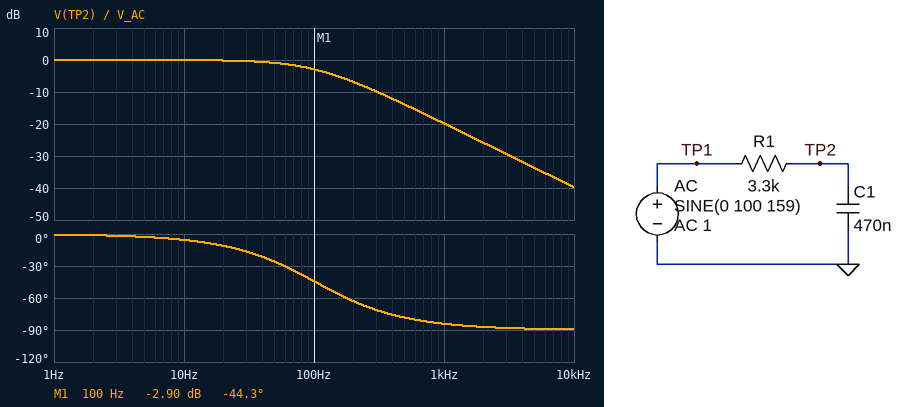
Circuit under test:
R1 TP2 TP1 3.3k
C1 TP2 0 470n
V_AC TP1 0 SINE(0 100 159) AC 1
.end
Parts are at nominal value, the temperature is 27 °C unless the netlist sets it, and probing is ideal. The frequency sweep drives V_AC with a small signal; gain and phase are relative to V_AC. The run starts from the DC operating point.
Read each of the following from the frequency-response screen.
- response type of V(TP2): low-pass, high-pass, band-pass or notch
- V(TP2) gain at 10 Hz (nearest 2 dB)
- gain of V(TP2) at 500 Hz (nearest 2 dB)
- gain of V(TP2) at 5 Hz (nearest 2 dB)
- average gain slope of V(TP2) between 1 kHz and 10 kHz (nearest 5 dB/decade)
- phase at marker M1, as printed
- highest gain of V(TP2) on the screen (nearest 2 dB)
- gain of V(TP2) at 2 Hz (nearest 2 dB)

low-pass
0 dB
-14 dB
0 dB
-20 dB/decade
-44.3 deg
0 dB
0 dB
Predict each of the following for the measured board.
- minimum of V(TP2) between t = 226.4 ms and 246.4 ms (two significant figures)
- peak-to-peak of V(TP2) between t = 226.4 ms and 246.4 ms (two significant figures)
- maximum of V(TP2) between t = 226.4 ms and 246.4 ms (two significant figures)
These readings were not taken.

-54 V
110 V
54 V
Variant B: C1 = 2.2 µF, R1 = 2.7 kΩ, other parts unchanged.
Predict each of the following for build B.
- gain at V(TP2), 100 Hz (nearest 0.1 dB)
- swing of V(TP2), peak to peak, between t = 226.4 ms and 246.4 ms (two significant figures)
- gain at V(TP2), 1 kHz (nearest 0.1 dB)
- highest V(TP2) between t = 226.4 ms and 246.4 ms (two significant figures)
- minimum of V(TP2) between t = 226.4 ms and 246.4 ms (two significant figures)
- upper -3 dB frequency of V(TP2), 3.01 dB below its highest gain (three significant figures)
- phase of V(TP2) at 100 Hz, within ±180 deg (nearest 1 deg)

-11.7 dB
33 V
-31.4 dB
17 V
-17 V
26.8 Hz
-75 deg
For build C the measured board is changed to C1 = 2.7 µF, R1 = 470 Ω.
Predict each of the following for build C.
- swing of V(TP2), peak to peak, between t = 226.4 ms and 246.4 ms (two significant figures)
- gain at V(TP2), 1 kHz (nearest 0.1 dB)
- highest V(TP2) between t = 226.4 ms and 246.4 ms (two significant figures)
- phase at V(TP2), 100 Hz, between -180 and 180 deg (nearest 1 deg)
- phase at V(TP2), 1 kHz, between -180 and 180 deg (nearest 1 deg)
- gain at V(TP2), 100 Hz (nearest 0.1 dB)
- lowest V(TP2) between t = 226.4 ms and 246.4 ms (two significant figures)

120 V
-18.1 dB
62 V
-39 deg
-83 deg
-2.1 dB
-62 V
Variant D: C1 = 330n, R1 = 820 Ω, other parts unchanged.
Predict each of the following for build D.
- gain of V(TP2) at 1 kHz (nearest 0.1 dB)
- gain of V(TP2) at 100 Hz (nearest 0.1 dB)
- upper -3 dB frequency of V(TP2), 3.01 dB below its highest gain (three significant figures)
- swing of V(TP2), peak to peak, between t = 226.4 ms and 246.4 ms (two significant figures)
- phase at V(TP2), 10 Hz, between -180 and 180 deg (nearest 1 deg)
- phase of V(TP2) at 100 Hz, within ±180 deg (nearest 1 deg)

-5.9 dB
-0.1 dB
588 Hz
190 V
-1 deg
-10 deg
